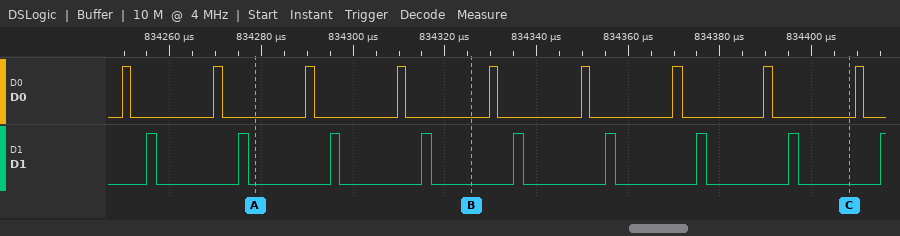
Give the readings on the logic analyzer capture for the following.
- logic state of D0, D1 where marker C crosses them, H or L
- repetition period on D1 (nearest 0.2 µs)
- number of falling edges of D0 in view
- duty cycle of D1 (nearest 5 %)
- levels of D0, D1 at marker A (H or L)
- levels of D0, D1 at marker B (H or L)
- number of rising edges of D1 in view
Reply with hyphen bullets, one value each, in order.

- D0=L, D1=L
- 20 µs
- 9
- 10 %
- D0=L, D1=L
- D0=L, D1=L
- 9
